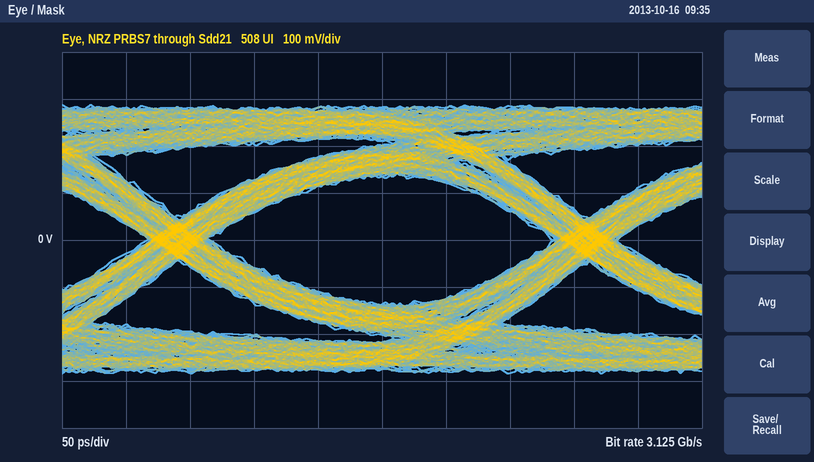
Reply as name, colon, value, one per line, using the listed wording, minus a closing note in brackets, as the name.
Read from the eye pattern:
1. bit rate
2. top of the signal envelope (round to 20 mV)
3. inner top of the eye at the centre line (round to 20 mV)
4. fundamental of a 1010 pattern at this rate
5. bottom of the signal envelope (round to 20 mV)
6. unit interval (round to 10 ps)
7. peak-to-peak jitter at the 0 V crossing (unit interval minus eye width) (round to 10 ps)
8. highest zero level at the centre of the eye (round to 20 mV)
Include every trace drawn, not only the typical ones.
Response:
bit rate: 3.125 Gb/s
top of the signal envelope: 280 mV
inner top of the eye at the centre line: 140 mV
fundamental of a 1010 pattern at this rate: 1.5625 GHz
bottom of the signal envelope: -280 mV
unit interval: 320 ps
peak-to-peak jitter at the 0 V crossing (unit interval minus eye width): 50 ps
highest zero level at the centre of the eye: -140 mV
